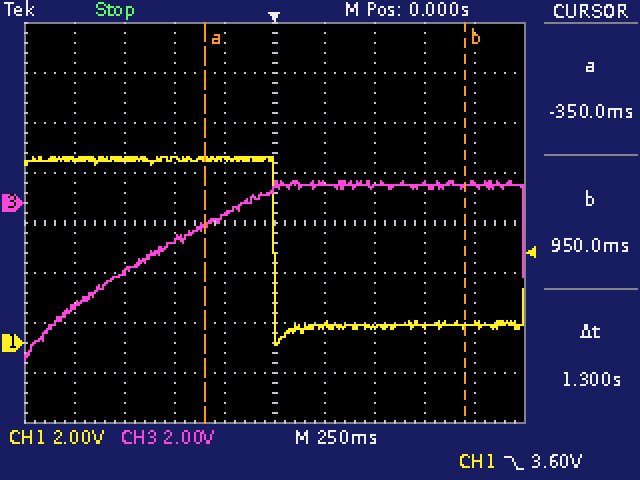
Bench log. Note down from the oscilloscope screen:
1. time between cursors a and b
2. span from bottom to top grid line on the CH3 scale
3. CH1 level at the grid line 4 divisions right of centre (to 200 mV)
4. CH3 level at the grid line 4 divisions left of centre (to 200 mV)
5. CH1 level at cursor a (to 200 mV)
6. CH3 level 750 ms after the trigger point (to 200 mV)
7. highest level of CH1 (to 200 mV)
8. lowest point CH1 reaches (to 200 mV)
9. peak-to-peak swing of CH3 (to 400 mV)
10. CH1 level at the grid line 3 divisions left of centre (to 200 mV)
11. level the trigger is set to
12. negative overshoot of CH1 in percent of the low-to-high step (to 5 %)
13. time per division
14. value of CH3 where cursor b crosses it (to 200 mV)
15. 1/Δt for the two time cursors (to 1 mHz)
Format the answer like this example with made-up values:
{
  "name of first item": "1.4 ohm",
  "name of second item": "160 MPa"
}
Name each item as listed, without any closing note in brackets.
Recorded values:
{
  "time between cursors a and b": "1.3 s",
  "span from bottom to top grid line on the CH3 scale": "16 V",
  "CH1 level at the grid line 4 divisions right of centre": "800 mV",
  "CH3 level at the grid line 4 divisions left of centre": "-4.2 V",
  "CH1 level at cursor a": "7.4 V",
  "CH3 level 750 ms after the trigger point": "800 mV",
  "highest level of CH1": "7.4 V",
  "lowest point CH1 reaches": "0.0 V",
  "peak-to-peak swing of CH3": "7.2 V",
  "CH1 level at the grid line 3 divisions left of centre": "7.4 V",
  "level the trigger is set to": "3.60 V",
  "negative overshoot of CH1 in percent of the low-to-high step": "10 %",
  "time per division": "250 ms",
  "value of CH3 where cursor b crosses it": "800 mV",
  "1/Δt for the two time cursors": "769 mHz"
}
